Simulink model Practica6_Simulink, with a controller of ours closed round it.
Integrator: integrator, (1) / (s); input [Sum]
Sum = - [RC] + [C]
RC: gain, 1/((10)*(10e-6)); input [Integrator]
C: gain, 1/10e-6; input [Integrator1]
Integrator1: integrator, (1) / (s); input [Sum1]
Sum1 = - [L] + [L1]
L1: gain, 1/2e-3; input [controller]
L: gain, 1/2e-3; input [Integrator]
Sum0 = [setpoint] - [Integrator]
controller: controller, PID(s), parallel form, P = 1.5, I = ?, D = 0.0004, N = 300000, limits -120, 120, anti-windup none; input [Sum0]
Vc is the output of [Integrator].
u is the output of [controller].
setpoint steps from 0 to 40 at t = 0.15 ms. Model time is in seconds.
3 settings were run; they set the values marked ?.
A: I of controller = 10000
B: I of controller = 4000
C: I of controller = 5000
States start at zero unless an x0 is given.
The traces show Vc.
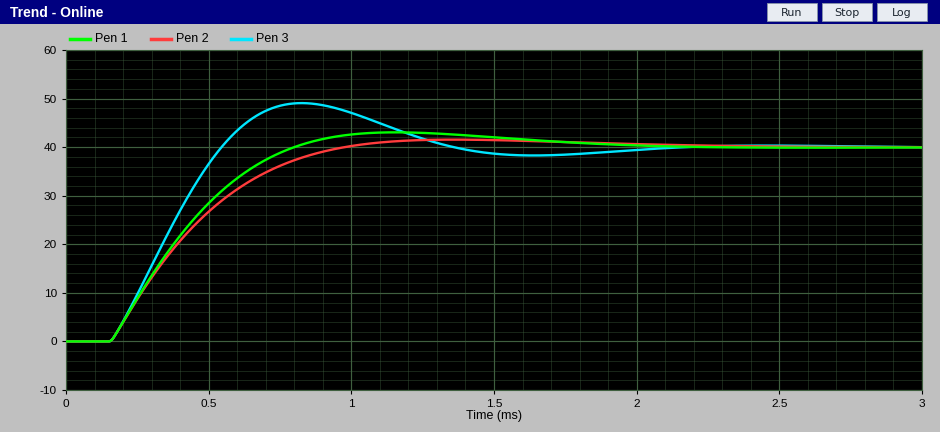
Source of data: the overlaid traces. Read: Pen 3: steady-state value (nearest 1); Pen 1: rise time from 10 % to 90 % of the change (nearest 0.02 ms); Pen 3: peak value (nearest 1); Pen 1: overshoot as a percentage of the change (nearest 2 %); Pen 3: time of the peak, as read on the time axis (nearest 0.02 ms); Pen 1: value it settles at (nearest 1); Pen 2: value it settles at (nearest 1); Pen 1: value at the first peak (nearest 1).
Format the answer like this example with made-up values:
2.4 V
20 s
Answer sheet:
40
0.46 ms
49
8 %
0.82 ms
40
40
43
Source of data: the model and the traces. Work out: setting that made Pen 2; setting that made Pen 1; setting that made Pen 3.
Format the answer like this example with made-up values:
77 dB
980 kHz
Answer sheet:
B
C
A
